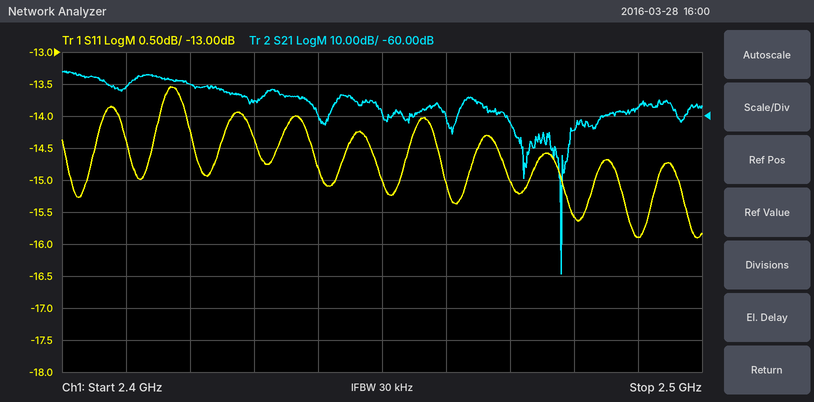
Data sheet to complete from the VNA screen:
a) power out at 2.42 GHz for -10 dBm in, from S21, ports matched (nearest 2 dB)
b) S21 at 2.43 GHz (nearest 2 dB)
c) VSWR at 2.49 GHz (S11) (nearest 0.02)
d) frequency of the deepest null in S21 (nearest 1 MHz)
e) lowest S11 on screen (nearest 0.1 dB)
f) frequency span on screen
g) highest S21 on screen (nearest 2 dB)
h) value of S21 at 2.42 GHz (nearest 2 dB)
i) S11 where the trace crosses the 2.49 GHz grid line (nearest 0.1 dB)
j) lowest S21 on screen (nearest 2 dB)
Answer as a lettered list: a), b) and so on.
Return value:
a) -60 dBm
b) -56 dB
c) 1.38
d) 2.478 GHz
e) -15.9 dB
f) 100 MHz
g) -46 dB
h) -50 dB
i) -15.9 dB
j) -110 dB
